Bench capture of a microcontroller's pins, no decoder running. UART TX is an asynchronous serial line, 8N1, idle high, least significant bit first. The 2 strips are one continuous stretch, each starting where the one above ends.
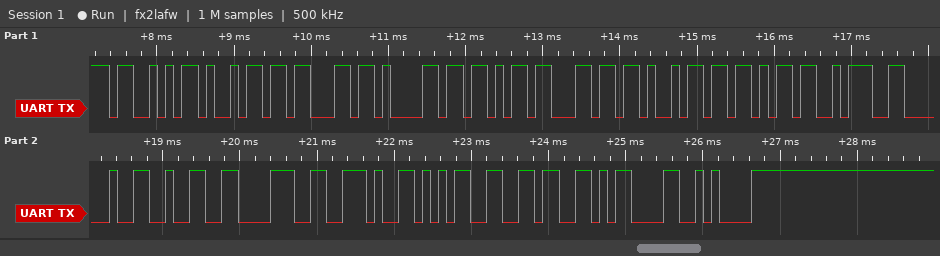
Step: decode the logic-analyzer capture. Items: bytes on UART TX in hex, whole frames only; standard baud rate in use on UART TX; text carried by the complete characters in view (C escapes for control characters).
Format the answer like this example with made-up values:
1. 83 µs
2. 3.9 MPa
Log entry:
1. 53 69 63 61 6B 6C 69 6B 3A 20 32 38 2E 35 36 0D 0A
2. 9600 baud
3. "Sicaklik: 28.56\r\n"
